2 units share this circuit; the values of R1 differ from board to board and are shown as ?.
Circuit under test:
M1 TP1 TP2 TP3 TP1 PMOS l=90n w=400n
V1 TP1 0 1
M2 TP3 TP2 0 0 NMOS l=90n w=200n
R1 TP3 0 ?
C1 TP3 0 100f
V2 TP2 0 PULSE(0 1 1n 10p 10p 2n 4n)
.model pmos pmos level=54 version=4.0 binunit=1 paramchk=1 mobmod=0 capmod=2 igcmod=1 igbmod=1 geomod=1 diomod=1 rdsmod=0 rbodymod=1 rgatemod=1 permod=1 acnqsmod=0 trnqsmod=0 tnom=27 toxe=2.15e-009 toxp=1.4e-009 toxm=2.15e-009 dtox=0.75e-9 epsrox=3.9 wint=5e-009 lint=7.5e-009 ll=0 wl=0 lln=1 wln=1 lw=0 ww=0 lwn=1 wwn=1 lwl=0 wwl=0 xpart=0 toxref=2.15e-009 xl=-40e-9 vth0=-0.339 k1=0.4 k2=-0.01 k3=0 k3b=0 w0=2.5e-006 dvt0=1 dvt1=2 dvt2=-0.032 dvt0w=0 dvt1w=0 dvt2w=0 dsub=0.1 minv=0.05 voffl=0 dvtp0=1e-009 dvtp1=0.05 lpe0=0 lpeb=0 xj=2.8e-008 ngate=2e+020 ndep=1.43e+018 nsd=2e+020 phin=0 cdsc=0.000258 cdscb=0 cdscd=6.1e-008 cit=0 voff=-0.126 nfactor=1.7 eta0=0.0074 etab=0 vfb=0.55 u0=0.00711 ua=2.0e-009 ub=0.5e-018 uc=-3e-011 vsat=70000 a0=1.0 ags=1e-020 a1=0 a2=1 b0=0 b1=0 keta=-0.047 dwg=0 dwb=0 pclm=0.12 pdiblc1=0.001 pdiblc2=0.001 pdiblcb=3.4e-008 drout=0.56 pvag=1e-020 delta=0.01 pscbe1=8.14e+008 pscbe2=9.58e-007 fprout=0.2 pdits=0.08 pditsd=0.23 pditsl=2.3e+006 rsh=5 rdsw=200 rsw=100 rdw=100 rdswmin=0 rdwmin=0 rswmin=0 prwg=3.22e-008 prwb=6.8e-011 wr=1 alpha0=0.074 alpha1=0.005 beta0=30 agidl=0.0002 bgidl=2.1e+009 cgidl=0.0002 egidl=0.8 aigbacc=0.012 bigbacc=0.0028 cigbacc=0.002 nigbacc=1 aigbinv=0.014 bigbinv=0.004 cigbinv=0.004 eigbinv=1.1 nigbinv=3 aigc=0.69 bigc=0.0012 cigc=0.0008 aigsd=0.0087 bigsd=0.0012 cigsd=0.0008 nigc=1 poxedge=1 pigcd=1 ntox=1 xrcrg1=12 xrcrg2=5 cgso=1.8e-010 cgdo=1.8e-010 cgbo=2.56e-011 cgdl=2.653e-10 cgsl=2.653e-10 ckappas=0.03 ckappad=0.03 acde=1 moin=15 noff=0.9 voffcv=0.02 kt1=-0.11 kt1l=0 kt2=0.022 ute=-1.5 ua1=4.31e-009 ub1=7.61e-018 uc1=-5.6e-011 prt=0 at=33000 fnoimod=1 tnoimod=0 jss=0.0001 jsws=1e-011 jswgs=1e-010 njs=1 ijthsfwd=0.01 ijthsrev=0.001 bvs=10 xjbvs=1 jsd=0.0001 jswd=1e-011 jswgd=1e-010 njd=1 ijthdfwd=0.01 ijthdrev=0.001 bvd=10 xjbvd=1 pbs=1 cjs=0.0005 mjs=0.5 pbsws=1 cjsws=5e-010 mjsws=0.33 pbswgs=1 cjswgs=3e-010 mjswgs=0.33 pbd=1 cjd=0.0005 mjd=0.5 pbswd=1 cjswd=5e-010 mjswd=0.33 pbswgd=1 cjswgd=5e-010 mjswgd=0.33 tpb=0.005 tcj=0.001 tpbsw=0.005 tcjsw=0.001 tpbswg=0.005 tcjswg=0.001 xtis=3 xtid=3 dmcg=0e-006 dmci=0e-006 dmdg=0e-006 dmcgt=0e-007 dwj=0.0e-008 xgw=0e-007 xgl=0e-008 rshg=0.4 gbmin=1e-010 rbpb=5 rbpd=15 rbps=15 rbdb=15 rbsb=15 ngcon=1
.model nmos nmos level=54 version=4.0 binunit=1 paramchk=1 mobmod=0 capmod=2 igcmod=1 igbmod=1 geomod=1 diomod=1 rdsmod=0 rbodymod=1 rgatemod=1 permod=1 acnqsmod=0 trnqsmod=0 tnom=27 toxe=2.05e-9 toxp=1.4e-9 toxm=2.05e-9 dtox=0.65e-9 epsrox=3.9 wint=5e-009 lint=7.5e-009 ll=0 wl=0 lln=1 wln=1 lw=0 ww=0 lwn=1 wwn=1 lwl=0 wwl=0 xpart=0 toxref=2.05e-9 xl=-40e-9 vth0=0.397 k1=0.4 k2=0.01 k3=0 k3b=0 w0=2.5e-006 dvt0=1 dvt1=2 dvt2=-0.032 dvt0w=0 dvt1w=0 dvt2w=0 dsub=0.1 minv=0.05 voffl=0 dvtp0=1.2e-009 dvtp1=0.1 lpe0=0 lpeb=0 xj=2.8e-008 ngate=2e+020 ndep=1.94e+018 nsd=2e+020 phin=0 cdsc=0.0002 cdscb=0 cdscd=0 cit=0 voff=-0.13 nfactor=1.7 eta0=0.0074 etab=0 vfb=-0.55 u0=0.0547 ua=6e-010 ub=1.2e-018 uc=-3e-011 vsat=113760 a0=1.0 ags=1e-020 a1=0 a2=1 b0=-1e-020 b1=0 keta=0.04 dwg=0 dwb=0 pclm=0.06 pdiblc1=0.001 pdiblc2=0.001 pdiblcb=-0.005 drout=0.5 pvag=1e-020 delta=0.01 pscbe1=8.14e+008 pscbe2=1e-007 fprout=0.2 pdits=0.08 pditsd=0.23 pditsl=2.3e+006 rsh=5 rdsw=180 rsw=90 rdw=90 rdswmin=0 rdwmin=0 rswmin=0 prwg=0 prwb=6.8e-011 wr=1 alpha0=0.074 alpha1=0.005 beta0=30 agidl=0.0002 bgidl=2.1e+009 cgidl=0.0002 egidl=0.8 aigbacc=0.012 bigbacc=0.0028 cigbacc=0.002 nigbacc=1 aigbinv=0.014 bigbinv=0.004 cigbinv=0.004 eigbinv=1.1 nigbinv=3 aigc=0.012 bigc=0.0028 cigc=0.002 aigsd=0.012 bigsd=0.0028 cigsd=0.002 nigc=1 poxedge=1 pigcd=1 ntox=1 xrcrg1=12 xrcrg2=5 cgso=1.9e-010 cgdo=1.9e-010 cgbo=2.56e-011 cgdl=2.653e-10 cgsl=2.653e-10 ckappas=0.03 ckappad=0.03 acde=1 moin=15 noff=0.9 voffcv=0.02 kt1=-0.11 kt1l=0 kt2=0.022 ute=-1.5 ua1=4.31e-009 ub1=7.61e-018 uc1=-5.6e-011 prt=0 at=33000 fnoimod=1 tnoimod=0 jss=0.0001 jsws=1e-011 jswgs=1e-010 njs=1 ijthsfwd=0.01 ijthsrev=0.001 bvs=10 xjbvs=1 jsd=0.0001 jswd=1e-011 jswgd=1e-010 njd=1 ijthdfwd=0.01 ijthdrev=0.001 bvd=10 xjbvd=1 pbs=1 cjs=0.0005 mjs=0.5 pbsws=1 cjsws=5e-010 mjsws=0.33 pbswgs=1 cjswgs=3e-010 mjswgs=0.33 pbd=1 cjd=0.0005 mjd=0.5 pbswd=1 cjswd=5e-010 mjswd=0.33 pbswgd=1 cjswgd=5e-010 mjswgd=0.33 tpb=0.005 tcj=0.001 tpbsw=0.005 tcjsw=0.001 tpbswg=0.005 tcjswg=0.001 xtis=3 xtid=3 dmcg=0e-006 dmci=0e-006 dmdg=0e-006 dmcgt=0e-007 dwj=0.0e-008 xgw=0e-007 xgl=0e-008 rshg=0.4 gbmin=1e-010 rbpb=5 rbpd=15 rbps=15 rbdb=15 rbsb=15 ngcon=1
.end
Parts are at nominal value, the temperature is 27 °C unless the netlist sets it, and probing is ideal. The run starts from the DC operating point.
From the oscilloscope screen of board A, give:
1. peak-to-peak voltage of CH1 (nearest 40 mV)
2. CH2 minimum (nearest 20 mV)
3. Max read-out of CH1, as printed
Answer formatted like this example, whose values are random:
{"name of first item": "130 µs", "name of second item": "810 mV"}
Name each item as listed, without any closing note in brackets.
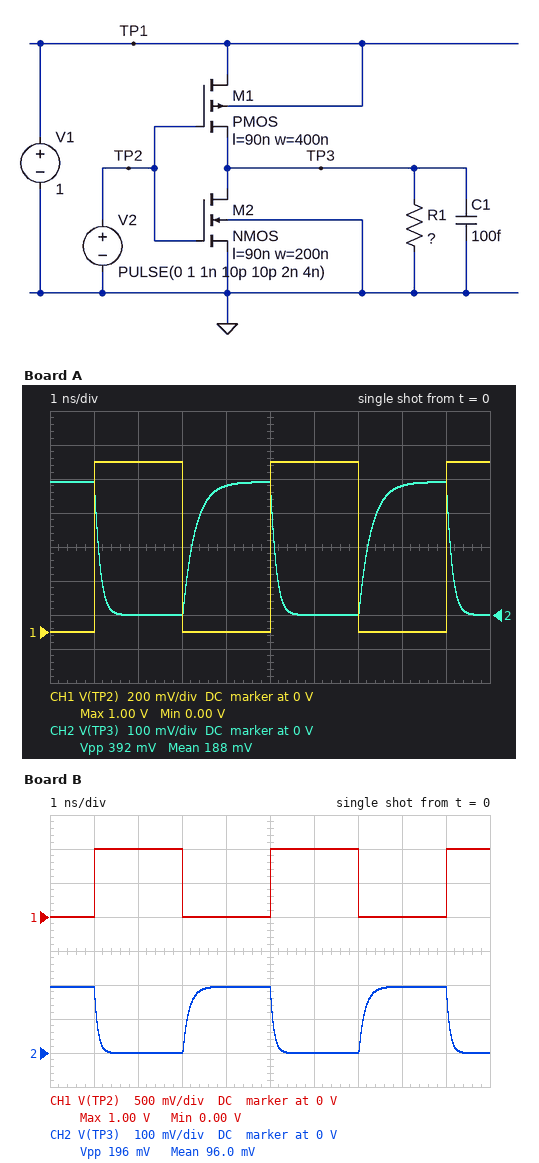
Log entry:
{"peak-to-peak voltage of CH1": "1.00 V", "CH2 minimum": "0 V", "Max read-out of CH1, as printed": "1.00 V"}
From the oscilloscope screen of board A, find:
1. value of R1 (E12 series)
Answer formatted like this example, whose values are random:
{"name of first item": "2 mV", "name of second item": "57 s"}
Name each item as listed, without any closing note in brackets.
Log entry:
{"value of R1": "3.3 kΩ"}
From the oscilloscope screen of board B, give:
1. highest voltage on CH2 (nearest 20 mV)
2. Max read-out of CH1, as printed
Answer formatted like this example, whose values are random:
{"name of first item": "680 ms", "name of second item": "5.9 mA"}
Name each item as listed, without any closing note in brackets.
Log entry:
{"highest voltage on CH2": "200 mV", "Max read-out of CH1, as printed": "1.00 V"}
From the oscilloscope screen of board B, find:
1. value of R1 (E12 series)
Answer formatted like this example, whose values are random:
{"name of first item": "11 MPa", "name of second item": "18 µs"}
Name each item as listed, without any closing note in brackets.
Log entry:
{"value of R1": "1.5 kΩ"}
